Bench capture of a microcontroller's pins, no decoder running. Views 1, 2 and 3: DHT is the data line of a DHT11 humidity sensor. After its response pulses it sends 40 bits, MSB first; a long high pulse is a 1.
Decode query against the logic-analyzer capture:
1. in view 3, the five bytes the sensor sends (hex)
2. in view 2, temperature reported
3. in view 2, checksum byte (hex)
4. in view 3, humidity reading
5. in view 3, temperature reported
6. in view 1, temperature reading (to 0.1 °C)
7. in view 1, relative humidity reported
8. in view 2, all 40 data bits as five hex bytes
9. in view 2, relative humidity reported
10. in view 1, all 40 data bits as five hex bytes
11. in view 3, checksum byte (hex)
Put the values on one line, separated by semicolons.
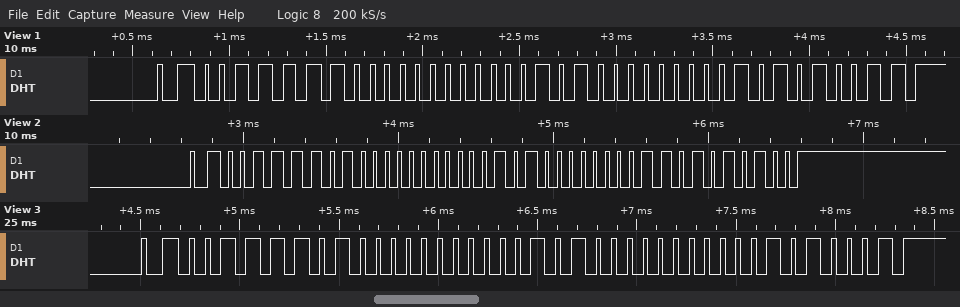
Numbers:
3D 00 14 00 51; 20.3 °C; 0x54; 61 %; 20.0 °C; 20.1 °C; 62 %; 3D 00 14 03 54; 61 %; 3E 00 14 01 53; 0x51
